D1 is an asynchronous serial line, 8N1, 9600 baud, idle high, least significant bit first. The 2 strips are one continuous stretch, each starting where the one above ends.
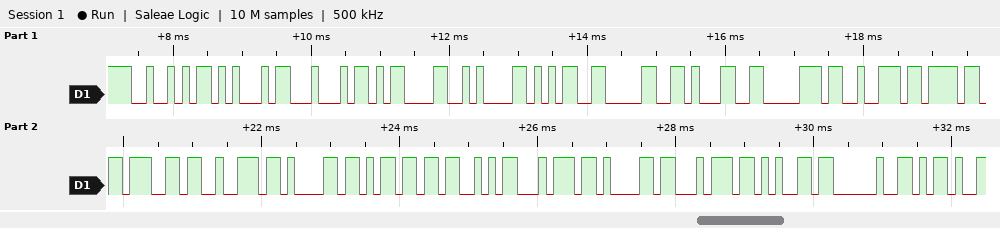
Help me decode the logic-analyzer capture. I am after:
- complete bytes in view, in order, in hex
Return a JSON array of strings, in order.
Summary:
["52 45 44 0D 0A 35 30 31 70 72 6F 67 72 61 6D 53 74 61 74 65 20 2D"]
